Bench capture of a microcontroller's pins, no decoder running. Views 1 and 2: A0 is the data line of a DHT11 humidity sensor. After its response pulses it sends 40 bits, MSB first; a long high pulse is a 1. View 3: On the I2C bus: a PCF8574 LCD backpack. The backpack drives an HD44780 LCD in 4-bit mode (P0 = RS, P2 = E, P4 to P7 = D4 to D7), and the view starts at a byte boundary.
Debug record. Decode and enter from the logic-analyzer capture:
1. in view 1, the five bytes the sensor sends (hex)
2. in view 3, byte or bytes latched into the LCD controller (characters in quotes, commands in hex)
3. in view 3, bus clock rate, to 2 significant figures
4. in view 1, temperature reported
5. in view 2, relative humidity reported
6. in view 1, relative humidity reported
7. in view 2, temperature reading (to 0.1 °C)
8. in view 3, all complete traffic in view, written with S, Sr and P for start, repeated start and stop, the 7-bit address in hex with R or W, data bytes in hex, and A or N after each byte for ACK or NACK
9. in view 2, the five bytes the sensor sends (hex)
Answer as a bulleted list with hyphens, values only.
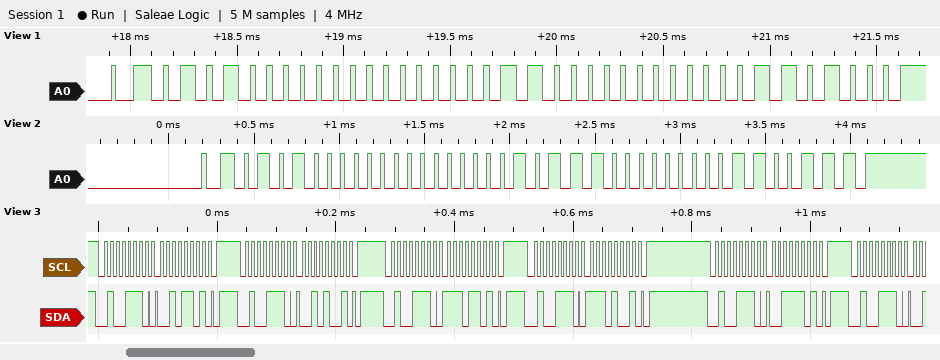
- 50 00 18 00 68
- '.'
- 100 kHz
- 24.0 °C
- 80 %
- 80 %
- 23.0 °C
- S 27W A 2D A P S 27W A 29 A P S 27W A ED A P S 27W A E9 A P S 27W A 3D A P S 27W A
- 50 00 17 00 67
